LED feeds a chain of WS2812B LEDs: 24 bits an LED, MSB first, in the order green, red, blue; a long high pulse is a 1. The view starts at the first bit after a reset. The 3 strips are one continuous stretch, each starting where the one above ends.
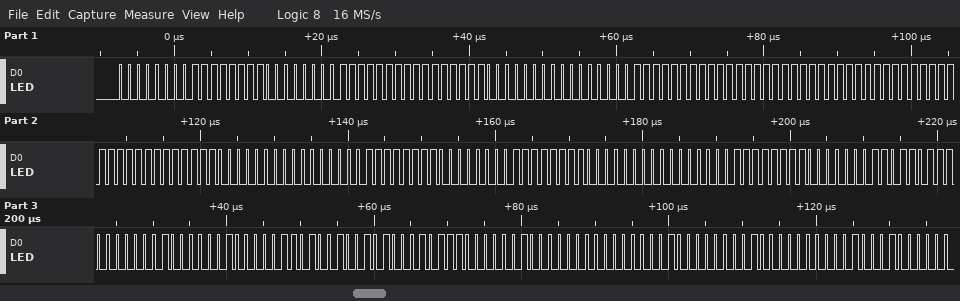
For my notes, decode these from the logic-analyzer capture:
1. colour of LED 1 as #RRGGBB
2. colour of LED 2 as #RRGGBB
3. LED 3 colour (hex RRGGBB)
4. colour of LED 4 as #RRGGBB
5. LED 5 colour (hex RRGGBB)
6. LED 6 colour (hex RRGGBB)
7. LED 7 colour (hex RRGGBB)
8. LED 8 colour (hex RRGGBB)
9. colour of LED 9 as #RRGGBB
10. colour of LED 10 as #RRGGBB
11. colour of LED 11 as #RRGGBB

#FF0000
#FFFF00
#FF00FF
#FFFFFF
#00FF00
#00FFFF
#0000FF
#B70101
#0D0225
#021700
#010200
